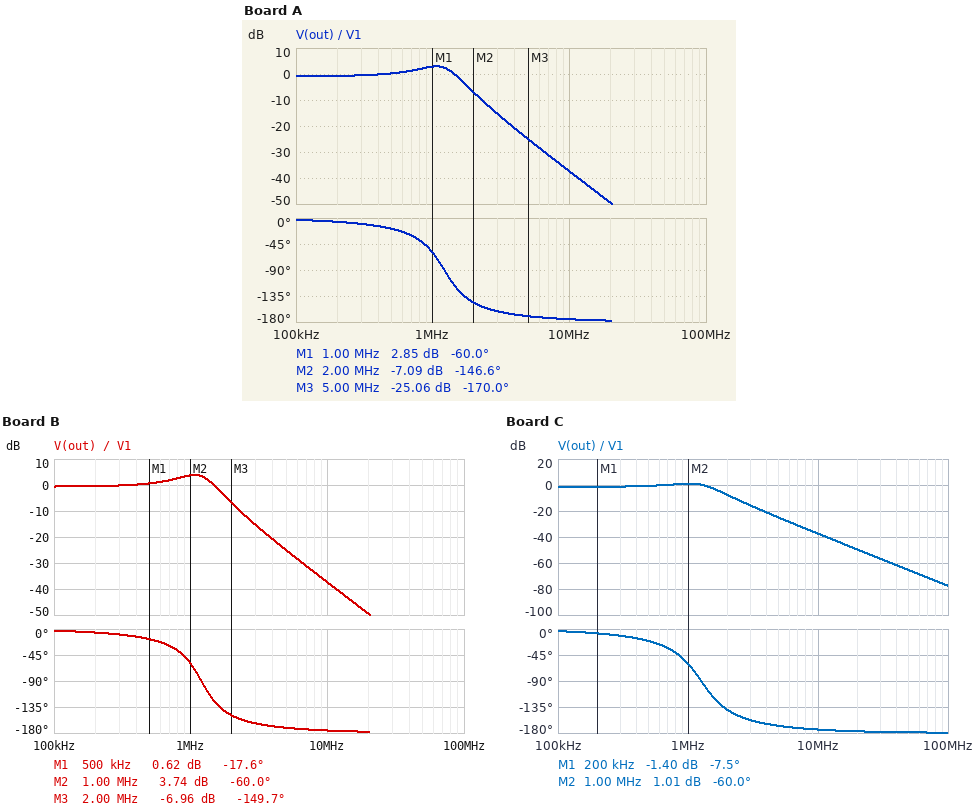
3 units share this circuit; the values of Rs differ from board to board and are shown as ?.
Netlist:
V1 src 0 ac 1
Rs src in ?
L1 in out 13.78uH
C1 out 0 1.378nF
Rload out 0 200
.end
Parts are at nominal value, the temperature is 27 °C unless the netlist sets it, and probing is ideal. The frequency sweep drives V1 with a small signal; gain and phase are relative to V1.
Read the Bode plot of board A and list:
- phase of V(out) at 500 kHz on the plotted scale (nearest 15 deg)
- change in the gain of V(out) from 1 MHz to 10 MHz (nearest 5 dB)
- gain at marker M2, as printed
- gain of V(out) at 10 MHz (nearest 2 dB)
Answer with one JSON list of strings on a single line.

["-15 deg", "-40 dB", "-7.09 dB", "-38 dB"]
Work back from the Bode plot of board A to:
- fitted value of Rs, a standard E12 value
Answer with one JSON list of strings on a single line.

["22 Ω"]
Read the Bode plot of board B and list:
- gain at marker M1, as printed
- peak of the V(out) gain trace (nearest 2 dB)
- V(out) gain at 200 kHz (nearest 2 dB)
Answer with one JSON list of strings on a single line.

["0.62 dB", "4 dB", "0 dB"]
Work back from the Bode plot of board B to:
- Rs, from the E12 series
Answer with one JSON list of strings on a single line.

["15 Ω"]
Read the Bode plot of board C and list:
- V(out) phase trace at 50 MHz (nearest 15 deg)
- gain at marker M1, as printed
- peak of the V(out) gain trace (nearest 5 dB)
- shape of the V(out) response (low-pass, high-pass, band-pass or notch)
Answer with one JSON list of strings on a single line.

["-180 deg", "-1.40 dB", "0 dB", "low-pass"]
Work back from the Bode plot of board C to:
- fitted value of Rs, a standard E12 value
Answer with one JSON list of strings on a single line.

["39 Ω"]
